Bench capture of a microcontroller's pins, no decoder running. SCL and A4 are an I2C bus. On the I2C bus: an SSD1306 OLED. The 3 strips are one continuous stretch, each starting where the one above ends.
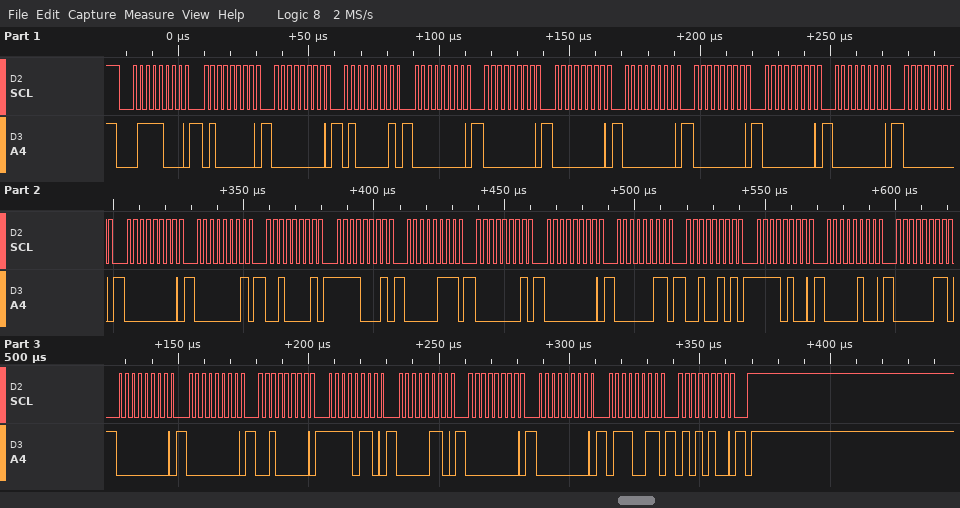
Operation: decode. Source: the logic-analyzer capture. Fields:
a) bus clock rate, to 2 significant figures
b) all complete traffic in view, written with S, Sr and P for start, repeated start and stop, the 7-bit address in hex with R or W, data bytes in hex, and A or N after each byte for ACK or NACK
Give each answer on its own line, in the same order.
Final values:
400 kHz
S 3CW A 40 A 00 A 41 A 00 A 00 A 00 A 00 A 00 A 00 A 00 A 00 A 00 A 01 A 21 A F1 A 07 A 01 A 00 A 03 A 25 A F4 A 04 A 03 A 00 A 00 A 20 A F6 A 06 A 00 A 00 A 73 A 54 A P
